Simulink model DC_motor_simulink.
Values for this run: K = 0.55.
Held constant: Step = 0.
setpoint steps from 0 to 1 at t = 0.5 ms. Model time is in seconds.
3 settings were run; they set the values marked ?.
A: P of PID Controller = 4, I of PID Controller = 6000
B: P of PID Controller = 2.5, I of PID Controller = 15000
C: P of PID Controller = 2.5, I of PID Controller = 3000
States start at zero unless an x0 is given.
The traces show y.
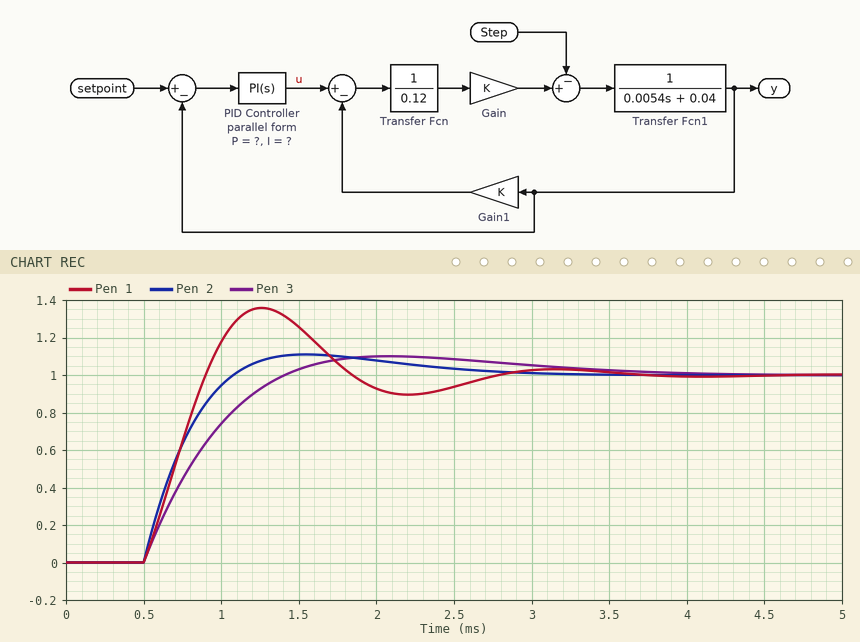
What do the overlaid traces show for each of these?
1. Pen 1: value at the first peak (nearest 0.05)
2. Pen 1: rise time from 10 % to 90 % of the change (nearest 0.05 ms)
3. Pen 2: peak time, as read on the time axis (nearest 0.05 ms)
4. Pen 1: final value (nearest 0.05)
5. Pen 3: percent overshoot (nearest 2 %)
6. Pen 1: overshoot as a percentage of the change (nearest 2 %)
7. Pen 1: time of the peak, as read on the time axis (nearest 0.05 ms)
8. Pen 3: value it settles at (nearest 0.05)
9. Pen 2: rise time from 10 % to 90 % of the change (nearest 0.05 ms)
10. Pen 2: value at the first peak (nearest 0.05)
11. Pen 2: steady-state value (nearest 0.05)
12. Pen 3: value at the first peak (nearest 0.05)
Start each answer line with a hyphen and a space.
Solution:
- 1.35
- 0.30 ms
- 1.55 ms
- 1.00
- 10 %
- 36 %
- 1.25 ms
- 1.00
- 0.40 ms
- 1.10
- 1.00
- 1.10
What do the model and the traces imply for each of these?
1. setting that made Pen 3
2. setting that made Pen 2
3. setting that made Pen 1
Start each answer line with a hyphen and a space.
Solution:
- C
- A
- B
